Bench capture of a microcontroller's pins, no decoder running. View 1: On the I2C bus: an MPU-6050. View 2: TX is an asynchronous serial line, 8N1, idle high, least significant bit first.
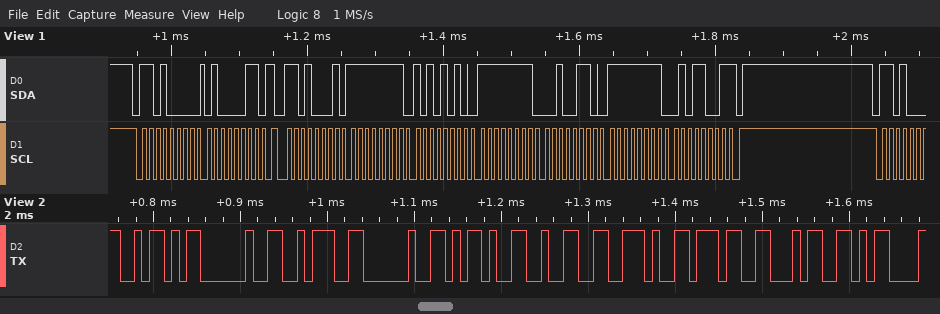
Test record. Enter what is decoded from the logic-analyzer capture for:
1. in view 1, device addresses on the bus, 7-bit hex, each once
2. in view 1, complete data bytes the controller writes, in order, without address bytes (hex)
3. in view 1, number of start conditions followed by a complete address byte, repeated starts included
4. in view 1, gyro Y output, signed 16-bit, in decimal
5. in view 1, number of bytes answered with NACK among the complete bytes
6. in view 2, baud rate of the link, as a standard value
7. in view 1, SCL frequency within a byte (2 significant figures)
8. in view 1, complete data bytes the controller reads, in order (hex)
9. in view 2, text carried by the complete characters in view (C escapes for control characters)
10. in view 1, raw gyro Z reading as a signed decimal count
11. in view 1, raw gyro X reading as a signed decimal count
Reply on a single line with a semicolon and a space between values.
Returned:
0x68; 43; 2; -218; 1; 115200 baud; 100 kHz; FF AA FF 26 FF 59; "Z : -2.74\r"; -167; -86
